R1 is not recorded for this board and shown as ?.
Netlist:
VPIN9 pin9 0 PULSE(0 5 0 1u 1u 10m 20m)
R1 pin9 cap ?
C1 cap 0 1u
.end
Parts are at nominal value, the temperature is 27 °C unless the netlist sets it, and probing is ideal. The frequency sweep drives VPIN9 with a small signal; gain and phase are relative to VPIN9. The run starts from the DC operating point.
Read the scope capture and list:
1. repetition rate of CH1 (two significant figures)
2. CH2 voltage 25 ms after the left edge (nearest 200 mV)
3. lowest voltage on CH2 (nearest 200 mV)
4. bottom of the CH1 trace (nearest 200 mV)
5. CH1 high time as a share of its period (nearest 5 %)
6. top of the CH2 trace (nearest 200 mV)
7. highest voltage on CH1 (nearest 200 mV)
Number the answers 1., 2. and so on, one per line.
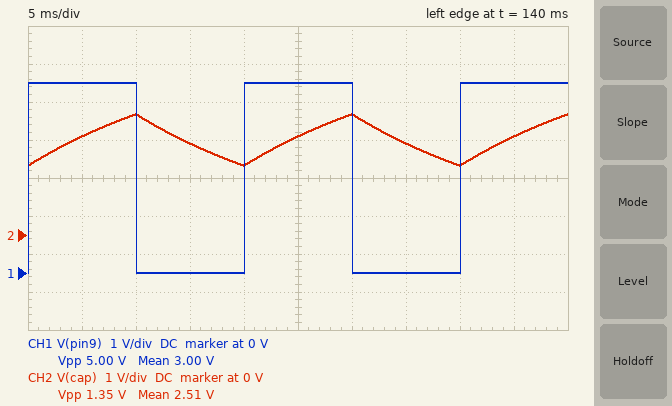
1. 50 Hz
2. 2.6 V
3. 1.8 V
4. 0 V
5. 50 %
6. 3.2 V
7. 5.0 V
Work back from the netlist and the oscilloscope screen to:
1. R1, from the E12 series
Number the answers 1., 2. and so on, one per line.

1. 18 kΩ
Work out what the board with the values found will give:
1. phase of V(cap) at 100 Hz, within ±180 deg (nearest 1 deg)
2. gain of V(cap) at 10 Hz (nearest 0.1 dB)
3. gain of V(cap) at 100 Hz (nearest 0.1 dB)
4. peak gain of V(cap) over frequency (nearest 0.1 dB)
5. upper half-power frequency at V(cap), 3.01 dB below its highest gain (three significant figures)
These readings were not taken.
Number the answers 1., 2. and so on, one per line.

1. -85 deg
2. -3.6 dB
3. -21.1 dB
4. 0 dB
5. 8.84 Hz
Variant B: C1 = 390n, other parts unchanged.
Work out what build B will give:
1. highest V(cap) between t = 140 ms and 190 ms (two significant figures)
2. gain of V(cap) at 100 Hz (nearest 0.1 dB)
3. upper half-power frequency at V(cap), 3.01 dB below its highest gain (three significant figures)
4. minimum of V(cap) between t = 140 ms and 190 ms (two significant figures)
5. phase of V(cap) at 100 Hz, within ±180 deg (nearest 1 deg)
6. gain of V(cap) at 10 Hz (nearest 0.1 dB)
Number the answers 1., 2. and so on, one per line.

1. 4.0 V
2. -13.1 dB
3. 22.7 Hz
4. 970 mV
5. -77 deg
6. -0.8 dB
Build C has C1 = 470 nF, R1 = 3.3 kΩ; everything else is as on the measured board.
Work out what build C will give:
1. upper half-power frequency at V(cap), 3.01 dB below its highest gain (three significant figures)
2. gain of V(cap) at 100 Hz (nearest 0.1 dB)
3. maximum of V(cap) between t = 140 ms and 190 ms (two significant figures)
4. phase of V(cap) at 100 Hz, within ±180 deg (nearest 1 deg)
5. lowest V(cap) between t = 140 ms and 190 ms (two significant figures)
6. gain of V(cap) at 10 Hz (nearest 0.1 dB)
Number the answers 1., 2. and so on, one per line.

1. 103 Hz
2. -2.9 dB
3. 5.0 V
4. -44 deg
5. 7.9 mV
6. 0 dB
